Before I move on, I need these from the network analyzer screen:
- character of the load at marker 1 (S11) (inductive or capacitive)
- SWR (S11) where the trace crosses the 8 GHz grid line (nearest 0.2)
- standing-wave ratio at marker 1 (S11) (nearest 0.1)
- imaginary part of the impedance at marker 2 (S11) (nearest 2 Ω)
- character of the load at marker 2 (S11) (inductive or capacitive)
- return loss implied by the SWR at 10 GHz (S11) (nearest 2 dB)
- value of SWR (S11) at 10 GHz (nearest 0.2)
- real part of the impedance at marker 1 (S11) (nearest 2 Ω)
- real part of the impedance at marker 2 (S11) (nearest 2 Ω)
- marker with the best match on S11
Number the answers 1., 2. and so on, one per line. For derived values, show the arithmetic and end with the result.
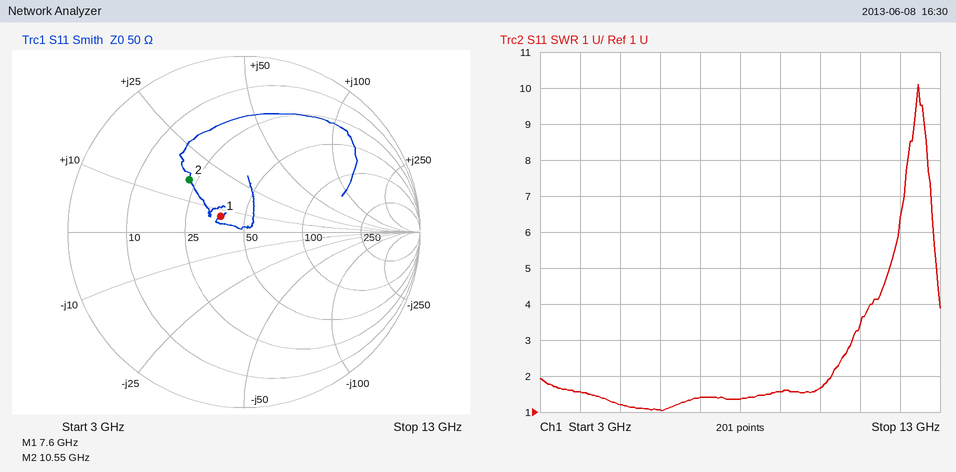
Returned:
1. inductive
2. 1.4
3. 1.4
4. +16 Ω
5. inductive
6. −20 log10((1.6 − 1)/(1.6 + 1)) ≈ 12.7 dB, so 12 dB to the nearest 2 dB
7. 1.6
8. 38 Ω
9. 22 Ω
10. marker 1
